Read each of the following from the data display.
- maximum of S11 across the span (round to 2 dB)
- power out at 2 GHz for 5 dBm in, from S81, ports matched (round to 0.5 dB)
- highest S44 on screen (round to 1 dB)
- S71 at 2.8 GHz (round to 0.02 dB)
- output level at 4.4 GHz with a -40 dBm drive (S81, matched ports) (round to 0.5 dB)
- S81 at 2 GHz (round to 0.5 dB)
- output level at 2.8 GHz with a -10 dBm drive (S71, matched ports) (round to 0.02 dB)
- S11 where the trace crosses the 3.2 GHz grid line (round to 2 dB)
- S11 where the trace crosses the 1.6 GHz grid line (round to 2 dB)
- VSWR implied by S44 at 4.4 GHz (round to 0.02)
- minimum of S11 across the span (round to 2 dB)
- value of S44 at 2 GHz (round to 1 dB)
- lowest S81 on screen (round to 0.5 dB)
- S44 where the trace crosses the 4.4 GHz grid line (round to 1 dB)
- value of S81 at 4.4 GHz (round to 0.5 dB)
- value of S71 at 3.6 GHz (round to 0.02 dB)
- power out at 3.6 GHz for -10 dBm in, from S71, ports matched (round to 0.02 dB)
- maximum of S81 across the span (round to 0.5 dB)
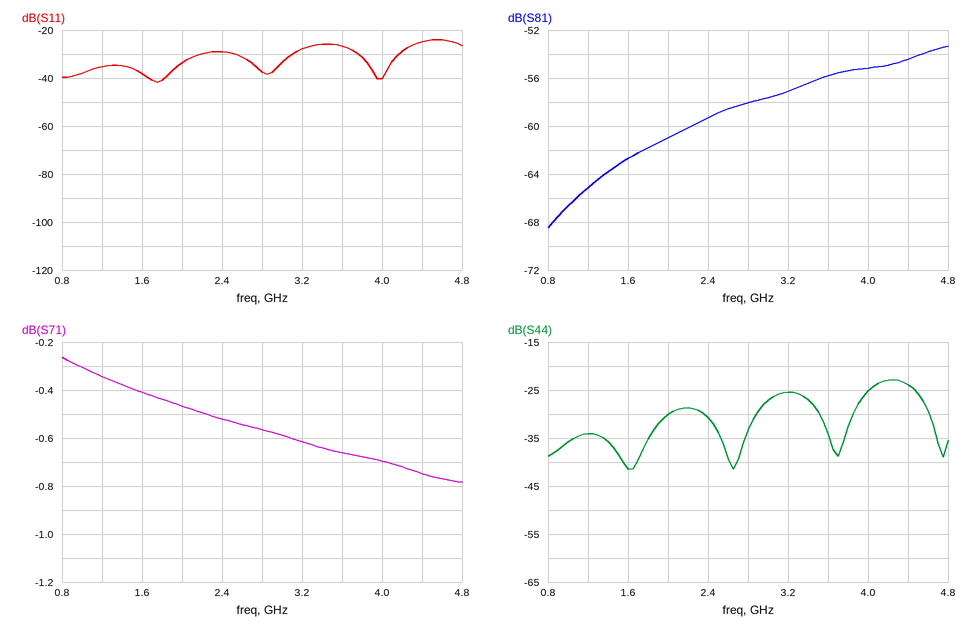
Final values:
-24 dB
-56.0 dBm
-23 dB
-0.56 dB
-94.5 dBm
-61.0 dB
-10.56 dBm
-28 dB
-38 dB
1.14
-42 dB
-30 dB
-68.5 dB
-24 dB
-54.5 dB
-0.66 dB
-10.66 dBm
-53.5 dB
